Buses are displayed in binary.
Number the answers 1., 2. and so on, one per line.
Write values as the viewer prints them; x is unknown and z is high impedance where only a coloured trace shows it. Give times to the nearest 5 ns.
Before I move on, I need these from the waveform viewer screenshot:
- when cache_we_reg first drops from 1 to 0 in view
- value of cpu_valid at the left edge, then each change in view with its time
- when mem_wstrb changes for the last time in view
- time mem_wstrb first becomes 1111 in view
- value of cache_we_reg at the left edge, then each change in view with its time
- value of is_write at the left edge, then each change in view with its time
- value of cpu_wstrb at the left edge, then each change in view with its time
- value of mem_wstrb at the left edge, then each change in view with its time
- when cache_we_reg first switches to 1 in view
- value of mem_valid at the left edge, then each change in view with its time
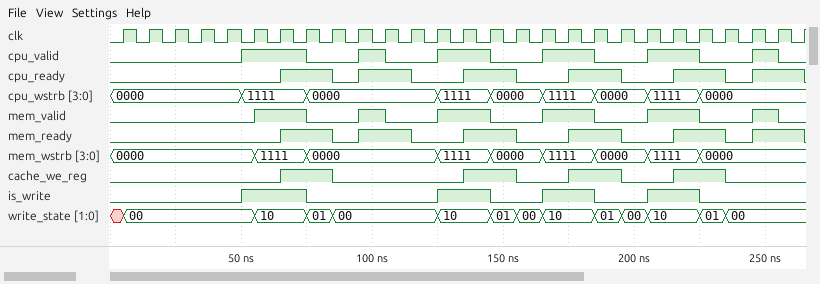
1. 85 ns
2. 0, 1 at 50 ns, 0 at 75 ns, 1 at 95 ns, 0 at 105 ns, 1 at 125 ns, 0 at 145 ns, 1 at 165 ns, 0 at 185 ns, 1 at 205 ns, 0 at 225 ns, 1 at 245 ns, 0 at 255 ns
3. 225 ns
4. 55 ns
5. 0, 1 at 65 ns, 0 at 85 ns, 1 at 135 ns, 0 at 155 ns, 1 at 175 ns, 0 at 195 ns, 1 at 215 ns, 0 at 235 ns
6. 0, 1 at 50 ns, 0 at 75 ns, 1 at 125 ns, 0 at 145 ns, 1 at 165 ns, 0 at 185 ns, 1 at 205 ns, 0 at 225 ns
7. 0000, 1111 at 50 ns, 0000 at 75 ns, 1111 at 125 ns, 0000 at 145 ns, 1111 at 165 ns, 0000 at 185 ns, 1111 at 205 ns, 0000 at 225 ns
8. 0000, 1111 at 55 ns, 0000 at 75 ns, 1111 at 125 ns, 0000 at 145 ns, 1111 at 165 ns, 0000 at 185 ns, 1111 at 205 ns, 0000 at 225 ns
9. 65 ns
10. 0, 1 at 55 ns, 0 at 75 ns, 1 at 95 ns, 0 at 105 ns, 1 at 125 ns, 0 at 145 ns, 1 at 165 ns, 0 at 185 ns, 1 at 205 ns, 0 at 225 ns, 1 at 245 ns, 0 at 255 ns
